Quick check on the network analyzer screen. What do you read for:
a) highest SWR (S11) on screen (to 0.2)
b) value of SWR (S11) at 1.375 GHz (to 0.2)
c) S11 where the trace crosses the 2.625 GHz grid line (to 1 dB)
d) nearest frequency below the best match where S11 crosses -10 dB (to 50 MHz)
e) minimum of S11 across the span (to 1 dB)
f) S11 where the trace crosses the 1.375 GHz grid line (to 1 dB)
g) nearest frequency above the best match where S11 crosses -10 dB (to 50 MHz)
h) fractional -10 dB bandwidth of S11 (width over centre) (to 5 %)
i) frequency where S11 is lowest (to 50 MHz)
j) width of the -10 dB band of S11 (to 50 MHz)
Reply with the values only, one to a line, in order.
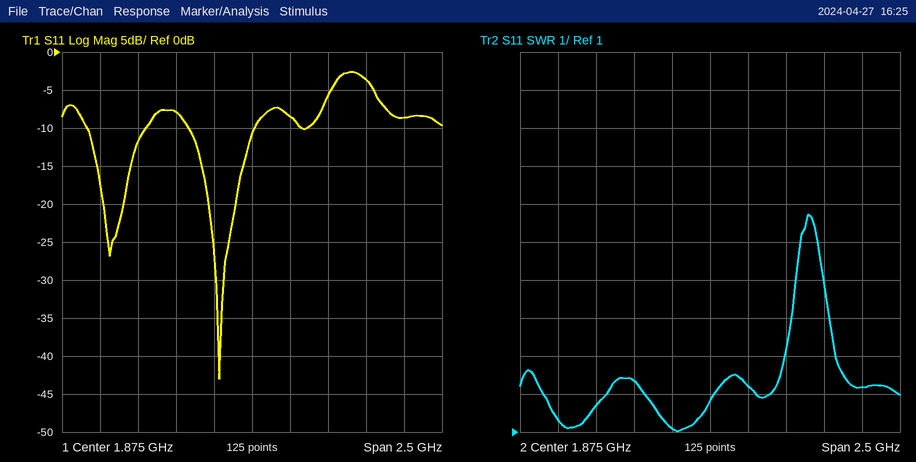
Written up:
6.8
2.4
-4 dB
1.45 GHz
-43 dB
-8 dB
1.90 GHz
25 %
1.65 GHz
450 MHz
